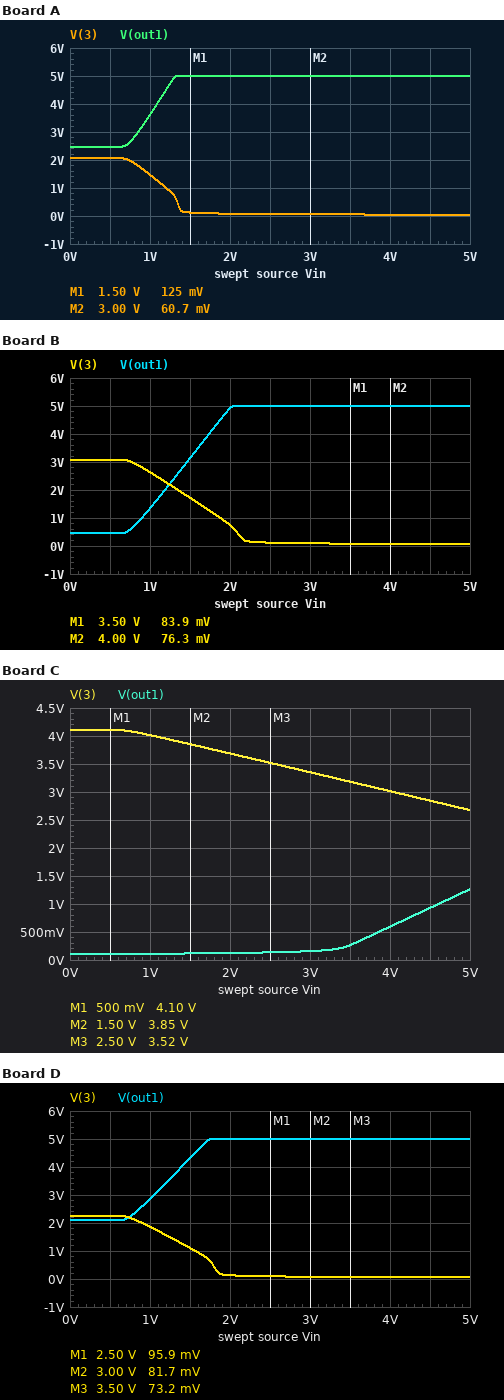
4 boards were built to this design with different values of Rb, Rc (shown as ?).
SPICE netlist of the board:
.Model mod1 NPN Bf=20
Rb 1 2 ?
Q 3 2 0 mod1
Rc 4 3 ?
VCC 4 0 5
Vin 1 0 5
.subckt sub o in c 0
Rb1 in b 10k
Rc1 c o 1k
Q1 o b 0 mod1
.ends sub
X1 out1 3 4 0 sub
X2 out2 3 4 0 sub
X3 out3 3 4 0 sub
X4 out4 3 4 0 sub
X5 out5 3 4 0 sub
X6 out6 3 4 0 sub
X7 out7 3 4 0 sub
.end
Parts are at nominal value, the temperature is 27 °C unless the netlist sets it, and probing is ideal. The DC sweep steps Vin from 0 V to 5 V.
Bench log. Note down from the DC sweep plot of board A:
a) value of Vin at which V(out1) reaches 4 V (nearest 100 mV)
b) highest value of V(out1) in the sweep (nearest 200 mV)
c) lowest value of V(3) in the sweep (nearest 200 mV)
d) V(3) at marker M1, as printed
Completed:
1.1 V
5.0 V
0 V
125 mV
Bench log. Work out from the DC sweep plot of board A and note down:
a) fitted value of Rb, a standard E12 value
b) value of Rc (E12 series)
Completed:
8.2 kΩ
3.3 kΩ
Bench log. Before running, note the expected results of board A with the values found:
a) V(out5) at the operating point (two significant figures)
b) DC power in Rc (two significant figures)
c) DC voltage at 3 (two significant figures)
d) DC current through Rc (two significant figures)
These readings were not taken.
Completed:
5.0 V
7.4 mW
45 mV
1.5 mA
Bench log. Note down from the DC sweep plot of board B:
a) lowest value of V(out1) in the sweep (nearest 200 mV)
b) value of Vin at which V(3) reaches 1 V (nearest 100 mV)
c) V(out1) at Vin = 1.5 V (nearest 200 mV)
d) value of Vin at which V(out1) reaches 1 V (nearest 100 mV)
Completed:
400 mV
1.9 V
3.2 V
900 mV
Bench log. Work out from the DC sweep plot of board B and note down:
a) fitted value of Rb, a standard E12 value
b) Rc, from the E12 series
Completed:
6.8 kΩ
1.2 kΩ
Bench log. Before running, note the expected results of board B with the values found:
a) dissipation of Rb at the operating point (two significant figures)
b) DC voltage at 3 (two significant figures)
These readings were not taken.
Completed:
2.6 mW
66 mV
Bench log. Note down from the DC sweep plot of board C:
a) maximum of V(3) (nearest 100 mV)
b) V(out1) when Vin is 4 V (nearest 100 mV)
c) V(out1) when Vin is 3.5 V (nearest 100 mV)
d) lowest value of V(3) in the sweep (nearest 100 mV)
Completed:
4.1 V
600 mV
300 mV
2.7 V
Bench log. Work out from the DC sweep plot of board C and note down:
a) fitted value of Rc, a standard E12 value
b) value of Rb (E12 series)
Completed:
390 Ω
18 kΩ
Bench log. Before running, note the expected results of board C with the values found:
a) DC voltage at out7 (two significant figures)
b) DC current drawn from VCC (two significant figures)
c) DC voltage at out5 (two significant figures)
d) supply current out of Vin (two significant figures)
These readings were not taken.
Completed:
1.3 V
32 mA
1.3 V
230 µA
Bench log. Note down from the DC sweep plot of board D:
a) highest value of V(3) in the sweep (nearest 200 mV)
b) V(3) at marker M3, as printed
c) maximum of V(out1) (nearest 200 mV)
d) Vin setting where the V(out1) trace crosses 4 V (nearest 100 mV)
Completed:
2.2 V
73.2 mV
5.0 V
1.4 V
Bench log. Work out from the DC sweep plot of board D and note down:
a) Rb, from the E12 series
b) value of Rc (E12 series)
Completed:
12 kΩ
2.7 kΩ
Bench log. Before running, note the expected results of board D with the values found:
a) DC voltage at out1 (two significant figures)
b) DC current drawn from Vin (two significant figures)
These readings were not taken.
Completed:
5.0 V
350 µA
